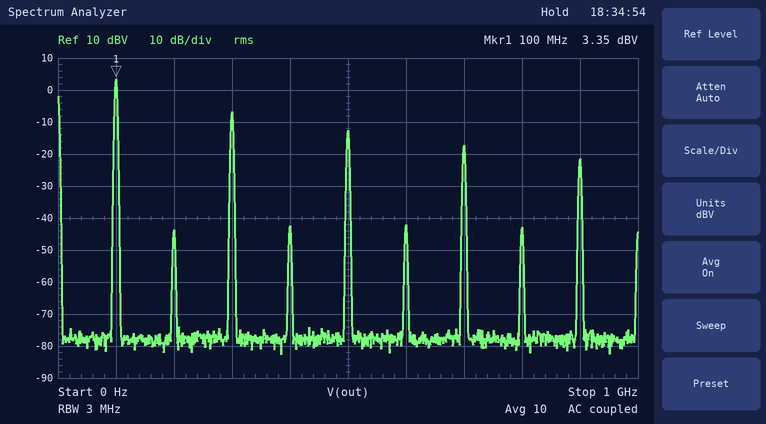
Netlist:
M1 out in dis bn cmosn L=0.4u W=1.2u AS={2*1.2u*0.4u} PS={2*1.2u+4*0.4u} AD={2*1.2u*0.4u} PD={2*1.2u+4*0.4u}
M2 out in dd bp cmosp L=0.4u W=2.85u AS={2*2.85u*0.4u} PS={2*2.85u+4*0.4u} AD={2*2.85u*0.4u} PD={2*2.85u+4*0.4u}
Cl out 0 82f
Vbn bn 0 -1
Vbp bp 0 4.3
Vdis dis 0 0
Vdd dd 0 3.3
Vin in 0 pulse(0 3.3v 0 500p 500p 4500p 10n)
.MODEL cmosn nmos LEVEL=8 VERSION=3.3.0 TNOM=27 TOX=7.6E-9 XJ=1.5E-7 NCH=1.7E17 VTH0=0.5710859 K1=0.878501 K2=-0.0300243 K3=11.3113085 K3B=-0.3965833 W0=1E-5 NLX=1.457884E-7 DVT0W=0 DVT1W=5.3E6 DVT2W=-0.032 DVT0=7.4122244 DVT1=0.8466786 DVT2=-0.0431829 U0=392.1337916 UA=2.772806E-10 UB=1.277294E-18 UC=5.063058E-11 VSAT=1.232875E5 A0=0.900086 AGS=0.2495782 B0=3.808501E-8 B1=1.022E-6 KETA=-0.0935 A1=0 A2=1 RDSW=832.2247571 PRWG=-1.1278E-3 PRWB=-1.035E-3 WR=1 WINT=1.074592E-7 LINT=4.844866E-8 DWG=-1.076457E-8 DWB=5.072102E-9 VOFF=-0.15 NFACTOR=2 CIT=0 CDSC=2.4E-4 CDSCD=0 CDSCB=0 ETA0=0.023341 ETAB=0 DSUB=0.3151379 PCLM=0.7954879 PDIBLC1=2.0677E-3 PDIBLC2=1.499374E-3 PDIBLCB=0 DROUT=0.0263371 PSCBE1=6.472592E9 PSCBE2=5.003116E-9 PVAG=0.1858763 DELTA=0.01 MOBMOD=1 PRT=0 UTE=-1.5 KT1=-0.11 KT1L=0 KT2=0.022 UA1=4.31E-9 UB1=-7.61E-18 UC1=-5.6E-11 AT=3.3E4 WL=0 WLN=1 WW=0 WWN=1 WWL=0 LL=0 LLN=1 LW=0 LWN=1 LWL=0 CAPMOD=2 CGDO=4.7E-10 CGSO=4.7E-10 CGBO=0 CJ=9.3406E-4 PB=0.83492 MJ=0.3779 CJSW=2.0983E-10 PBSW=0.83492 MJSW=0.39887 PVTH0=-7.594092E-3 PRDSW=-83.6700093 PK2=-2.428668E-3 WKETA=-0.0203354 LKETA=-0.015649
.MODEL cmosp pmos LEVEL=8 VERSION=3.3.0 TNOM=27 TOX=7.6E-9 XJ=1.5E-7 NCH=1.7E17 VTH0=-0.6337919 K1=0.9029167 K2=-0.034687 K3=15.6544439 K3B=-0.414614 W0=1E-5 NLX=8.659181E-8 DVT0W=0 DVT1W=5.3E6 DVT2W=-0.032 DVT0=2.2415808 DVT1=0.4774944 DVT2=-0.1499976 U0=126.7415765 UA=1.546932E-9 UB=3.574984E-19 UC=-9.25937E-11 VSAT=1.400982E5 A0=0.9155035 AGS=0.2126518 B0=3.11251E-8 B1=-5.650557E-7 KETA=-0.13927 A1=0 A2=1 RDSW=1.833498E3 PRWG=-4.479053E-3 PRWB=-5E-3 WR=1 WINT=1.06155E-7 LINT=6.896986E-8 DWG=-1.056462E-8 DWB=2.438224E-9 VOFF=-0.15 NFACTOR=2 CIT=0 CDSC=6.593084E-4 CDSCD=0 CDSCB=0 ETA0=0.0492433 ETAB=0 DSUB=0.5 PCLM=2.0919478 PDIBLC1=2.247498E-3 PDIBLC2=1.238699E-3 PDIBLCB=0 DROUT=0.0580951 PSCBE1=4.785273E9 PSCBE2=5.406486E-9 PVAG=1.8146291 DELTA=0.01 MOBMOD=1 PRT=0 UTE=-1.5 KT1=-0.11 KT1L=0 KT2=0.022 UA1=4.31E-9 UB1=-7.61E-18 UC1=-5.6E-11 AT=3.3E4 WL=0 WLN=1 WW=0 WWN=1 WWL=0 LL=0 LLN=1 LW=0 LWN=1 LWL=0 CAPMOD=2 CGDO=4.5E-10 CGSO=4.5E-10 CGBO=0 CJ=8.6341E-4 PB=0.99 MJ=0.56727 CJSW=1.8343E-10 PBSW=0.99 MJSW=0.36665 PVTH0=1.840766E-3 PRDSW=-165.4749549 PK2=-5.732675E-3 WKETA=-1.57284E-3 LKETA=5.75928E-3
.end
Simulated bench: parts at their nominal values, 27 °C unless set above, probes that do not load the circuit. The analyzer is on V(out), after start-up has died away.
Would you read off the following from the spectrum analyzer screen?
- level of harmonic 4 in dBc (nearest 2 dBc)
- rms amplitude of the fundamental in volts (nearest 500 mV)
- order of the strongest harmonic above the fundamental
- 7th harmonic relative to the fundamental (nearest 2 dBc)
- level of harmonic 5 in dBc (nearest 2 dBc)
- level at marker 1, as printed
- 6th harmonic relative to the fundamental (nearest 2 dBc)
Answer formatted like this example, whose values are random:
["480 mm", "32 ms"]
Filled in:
["-46 dBc", "1.5 V", "3", "-20 dBc", "-16 dBc", "3.35 dBV", "-46 dBc"]
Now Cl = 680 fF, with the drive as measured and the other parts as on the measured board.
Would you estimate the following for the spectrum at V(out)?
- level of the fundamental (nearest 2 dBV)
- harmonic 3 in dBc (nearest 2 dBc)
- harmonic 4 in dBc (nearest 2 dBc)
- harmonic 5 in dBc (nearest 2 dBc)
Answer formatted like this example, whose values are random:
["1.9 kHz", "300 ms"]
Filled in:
["0 dBV", "-22 dBc", "-50 dBc", "-30 dBc"]
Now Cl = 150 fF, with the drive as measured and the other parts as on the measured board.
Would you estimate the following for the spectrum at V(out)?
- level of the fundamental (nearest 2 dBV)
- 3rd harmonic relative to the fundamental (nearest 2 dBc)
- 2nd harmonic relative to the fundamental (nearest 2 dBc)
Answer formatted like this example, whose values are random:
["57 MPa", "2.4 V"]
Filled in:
["4 dBV", "-12 dBc", "-42 dBc"]
